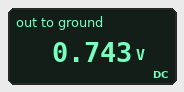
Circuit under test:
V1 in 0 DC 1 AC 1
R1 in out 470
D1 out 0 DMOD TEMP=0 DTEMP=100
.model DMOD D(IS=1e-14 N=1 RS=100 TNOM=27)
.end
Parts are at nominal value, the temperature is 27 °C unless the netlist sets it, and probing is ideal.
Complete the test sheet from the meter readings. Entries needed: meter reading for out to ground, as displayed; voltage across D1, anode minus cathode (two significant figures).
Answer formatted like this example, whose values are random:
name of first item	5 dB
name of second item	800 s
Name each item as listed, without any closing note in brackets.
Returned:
meter reading for out to ground, as displayed	0.743 V
voltage across D1, anode minus cathode	740 mV
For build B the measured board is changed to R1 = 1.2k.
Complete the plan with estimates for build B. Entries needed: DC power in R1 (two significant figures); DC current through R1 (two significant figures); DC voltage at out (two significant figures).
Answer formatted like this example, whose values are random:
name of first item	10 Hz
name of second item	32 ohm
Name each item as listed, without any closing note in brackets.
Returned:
DC power in R1	77 µW
DC current through R1	250 µA
DC voltage at out	700 mV
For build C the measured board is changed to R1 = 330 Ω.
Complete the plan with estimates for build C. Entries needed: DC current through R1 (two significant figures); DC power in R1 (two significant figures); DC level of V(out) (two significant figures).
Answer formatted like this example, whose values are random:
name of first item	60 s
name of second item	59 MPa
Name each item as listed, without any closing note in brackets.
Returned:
DC current through R1	710 µA
DC power in R1	170 µW
DC level of V(out)	770 mV
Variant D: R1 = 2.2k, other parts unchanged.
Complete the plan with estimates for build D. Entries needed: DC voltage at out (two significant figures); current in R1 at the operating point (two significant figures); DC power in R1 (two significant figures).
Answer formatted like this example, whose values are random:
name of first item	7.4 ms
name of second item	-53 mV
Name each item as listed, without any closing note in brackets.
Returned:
DC voltage at out	670 mV
current in R1 at the operating point	150 µA
DC power in R1	49 µW
